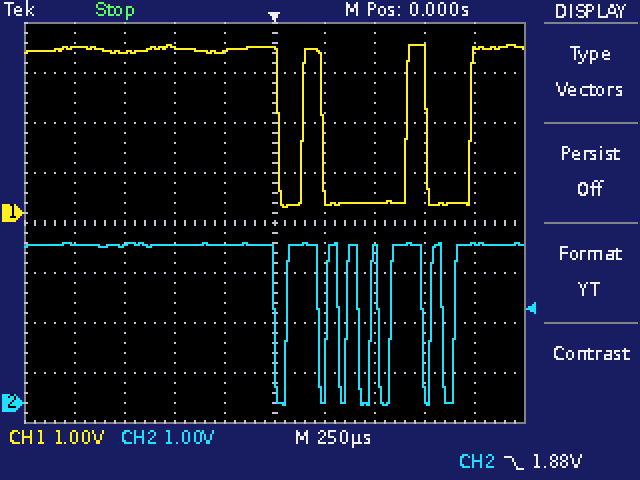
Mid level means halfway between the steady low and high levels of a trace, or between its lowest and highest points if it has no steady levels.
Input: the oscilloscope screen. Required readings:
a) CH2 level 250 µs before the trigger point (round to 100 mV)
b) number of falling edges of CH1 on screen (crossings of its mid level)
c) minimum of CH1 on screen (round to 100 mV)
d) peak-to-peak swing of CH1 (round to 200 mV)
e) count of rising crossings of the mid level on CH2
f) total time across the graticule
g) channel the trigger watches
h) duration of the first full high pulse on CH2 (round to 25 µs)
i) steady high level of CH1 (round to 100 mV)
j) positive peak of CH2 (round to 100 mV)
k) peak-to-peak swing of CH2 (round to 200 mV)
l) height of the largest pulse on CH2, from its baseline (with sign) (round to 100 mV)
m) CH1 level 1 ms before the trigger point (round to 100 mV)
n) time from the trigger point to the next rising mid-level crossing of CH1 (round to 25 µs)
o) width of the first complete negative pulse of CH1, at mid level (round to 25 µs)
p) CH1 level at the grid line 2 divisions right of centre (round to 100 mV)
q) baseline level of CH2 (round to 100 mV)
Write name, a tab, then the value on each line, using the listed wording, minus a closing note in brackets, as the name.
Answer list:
CH2 level 250 µs before the trigger point	3.2 V
number of falling edges of CH1 on screen	3
minimum of CH1 on screen	100 mV
peak-to-peak swing of CH1	3.2 V
count of rising crossings of the mid level on CH2	7
total time across the graticule	2.5 ms
channel the trigger watches	CH2
duration of the first full high pulse on CH2	150 µs
steady high level of CH1	3.3 V
positive peak of CH2	3.2 V
peak-to-peak swing of CH2	3.2 V
height of the largest pulse on CH2, from its baseline (with sign)	-3.2 V
CH1 level 1 ms before the trigger point	3.3 V
time from the trigger point to the next rising mid-level crossing of CH1	150 µs
width of the first complete negative pulse of CH1, at mid level	125 µs
CH1 level at the grid line 2 divisions right of centre	200 mV
baseline level of CH2	3.2 V
